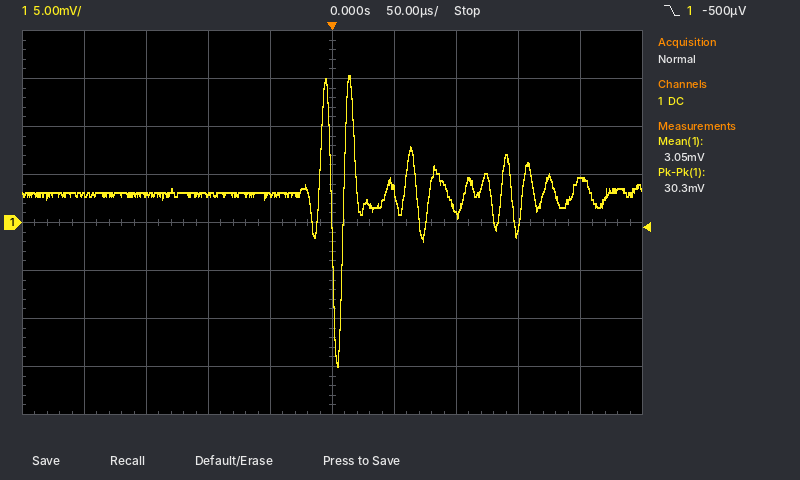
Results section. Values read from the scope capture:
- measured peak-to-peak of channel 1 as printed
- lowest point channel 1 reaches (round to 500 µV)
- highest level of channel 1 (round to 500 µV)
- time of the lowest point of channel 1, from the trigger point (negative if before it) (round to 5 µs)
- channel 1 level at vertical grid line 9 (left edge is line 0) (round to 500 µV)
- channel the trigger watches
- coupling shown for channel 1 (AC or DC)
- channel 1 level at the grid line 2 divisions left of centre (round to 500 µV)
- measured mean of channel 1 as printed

30.3 mV
-15.0 mV
15.5 mV
+5 µs
4.5 mV
channel 1
DC
3.0 mV
3.05 mV
